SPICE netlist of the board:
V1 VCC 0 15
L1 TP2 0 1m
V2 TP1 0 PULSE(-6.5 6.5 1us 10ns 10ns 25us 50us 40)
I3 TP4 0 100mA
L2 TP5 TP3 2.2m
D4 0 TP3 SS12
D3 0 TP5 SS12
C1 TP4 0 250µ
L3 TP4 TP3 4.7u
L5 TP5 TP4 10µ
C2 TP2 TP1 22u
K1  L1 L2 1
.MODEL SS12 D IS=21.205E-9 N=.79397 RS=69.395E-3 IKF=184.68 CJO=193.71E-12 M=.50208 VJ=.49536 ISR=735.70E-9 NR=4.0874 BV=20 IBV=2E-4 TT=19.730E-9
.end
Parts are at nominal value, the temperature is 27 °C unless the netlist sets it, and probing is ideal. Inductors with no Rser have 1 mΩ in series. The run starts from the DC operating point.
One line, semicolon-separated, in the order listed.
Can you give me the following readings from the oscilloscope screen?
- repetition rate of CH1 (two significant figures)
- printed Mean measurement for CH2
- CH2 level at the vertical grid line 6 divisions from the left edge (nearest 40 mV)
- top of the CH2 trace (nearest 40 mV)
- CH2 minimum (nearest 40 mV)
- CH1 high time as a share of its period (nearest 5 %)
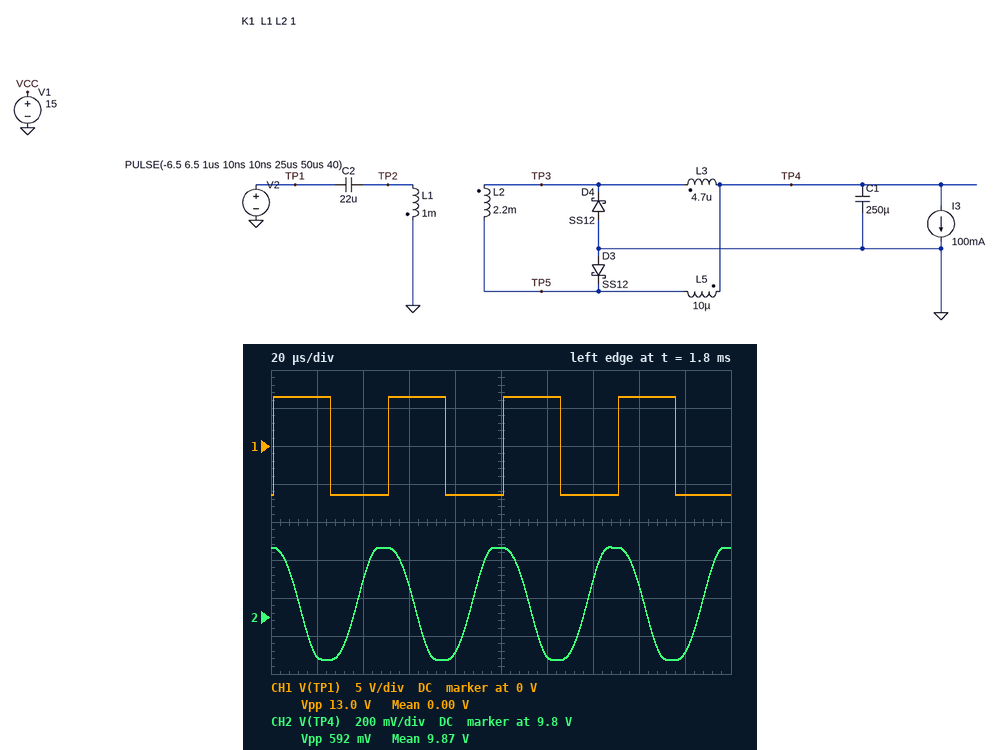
20 kHz; 9.87 V; 9.60 V; 10.16 V; 9.56 V; 50 %
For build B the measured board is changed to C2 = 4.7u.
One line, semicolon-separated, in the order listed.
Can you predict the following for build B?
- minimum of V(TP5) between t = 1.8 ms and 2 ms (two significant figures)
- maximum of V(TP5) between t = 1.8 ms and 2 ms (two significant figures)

-510 mV; 20 V
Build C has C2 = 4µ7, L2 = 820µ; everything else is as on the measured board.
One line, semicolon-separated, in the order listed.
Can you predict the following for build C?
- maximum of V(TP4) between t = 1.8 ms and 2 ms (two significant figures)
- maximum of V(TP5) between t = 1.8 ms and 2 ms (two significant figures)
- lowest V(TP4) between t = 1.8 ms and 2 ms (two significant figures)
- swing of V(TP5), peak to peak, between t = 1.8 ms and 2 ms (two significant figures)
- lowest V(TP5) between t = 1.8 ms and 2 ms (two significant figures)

9.9 V; 22 V; 9.7 V; 24 V; -2.2 V
